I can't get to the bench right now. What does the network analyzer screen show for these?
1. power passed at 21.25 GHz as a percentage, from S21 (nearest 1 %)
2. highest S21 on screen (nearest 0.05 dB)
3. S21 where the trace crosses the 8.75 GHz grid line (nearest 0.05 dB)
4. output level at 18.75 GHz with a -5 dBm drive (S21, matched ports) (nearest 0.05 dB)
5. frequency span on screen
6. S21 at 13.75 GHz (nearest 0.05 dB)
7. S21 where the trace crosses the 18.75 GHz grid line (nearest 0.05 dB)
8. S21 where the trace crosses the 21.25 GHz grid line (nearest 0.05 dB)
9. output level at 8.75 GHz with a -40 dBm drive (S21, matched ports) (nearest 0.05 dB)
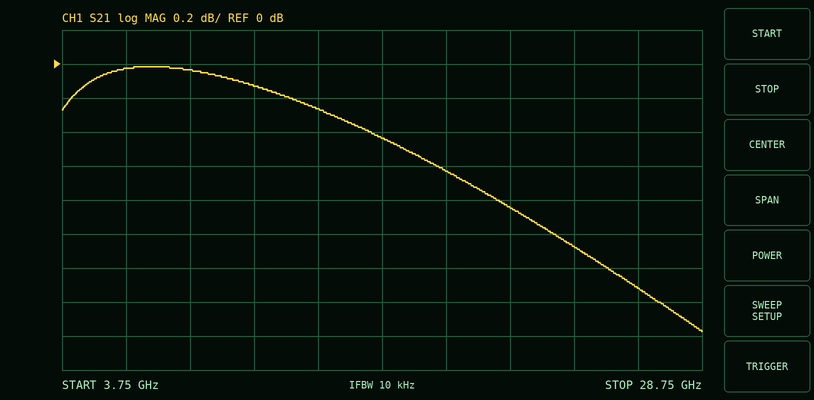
82 %
0.00 dB
-0.05 dB
-5.65 dBm
25 GHz
-0.25 dB
-0.65 dB
-0.85 dB
-40.05 dBm
